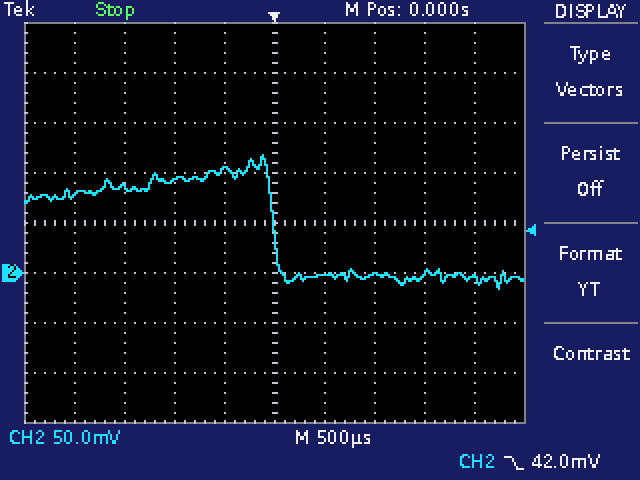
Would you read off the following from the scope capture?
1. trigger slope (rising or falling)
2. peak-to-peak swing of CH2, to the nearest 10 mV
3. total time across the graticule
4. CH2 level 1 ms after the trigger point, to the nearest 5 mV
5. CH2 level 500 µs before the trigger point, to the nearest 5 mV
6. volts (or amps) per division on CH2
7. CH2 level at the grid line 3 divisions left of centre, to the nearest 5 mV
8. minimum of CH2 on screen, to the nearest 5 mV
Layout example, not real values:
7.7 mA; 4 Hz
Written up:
falling; 130 mV; 5 ms; 0 mV; 105 mV; 50 mV; 85 mV; -15 mV
